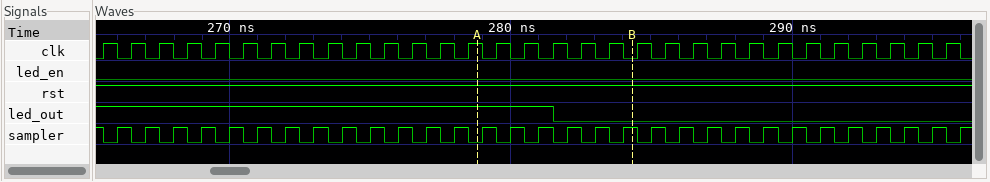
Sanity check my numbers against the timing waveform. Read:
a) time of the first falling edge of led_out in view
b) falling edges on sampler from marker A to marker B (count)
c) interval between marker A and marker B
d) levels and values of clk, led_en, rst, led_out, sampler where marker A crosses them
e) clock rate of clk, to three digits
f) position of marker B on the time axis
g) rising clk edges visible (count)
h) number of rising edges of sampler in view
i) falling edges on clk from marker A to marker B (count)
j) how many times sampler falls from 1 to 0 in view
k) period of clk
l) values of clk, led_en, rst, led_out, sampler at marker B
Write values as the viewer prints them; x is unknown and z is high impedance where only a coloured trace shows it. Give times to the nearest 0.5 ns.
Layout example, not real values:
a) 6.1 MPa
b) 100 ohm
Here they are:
a) 281.5 ns
b) 5
c) 5.5 ns
d) clk=1, led_en=0, rst=1, led_out=1, sampler=0
e) 1.00 GHz
f) 284.5 ns
g) 31
h) 31
i) 6
j) 31
k) 1 ns
l) clk=0, led_en=0, rst=1, led_out=0, sampler=1
